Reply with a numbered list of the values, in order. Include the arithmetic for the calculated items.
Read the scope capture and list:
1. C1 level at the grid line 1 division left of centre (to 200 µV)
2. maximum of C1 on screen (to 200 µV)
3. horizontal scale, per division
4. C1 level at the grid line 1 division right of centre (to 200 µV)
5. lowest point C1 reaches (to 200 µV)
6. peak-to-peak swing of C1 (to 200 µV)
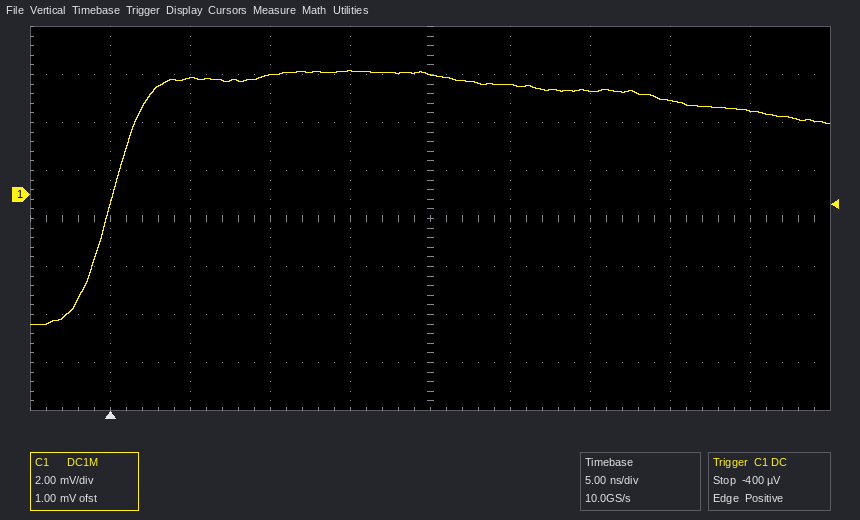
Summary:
1. 5.2 mV
2. 5.2 mV
3. 5 ns
4. 4.6 mV
5. -5.4 mV
6. 5.2 mV − (-5.4 mV) = 10.6 mV
